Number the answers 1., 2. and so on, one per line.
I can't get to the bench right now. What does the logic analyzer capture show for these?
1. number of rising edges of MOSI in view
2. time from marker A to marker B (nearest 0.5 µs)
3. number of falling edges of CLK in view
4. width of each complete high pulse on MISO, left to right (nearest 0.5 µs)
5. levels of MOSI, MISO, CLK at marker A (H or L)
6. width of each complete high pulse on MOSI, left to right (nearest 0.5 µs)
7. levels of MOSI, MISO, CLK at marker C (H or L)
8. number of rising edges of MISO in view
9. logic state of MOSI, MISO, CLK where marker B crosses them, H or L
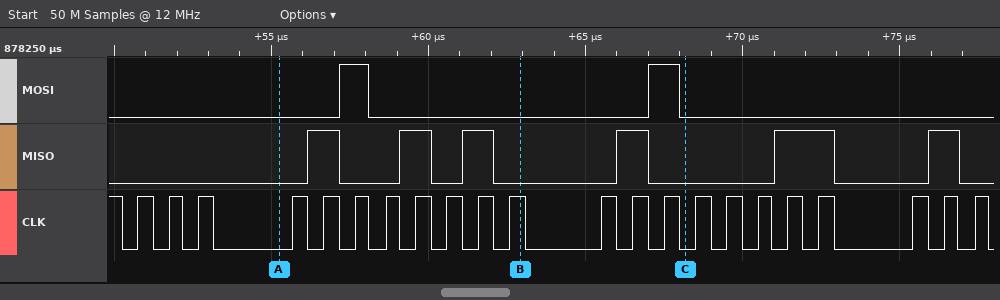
1. 2
2. 7.5 µs
3. 23
4. 1 µs, 1 µs, 1 µs, 1 µs, 2 µs, 1 µs
5. MOSI=L, MISO=L, CLK=L
6. 1 µs, 1 µs
7. MOSI=L, MISO=L, CLK=L
8. 6
9. MOSI=L, MISO=L, CLK=H
